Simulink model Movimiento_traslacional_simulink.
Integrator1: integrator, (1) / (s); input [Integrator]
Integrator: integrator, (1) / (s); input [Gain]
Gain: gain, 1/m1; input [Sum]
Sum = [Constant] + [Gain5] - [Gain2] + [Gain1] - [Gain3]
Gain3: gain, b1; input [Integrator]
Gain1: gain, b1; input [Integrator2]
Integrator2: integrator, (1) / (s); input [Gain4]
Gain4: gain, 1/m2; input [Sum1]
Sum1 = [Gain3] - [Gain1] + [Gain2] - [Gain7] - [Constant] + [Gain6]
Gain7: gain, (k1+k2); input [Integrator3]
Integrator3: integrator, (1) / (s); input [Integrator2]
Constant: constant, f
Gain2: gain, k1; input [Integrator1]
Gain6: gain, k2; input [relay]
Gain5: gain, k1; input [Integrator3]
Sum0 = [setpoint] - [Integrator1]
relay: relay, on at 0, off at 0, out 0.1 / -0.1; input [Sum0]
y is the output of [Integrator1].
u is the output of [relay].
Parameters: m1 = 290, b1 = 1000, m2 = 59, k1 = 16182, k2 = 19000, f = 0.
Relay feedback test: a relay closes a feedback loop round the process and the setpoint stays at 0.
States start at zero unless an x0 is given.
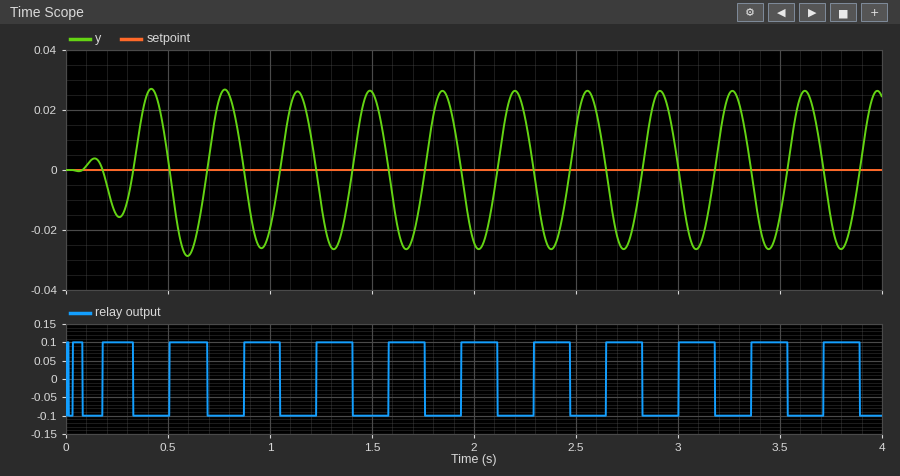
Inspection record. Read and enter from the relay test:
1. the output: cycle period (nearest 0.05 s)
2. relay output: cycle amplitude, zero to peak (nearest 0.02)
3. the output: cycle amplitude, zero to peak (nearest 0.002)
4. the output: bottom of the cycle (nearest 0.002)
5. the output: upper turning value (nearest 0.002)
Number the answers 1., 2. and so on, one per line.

1. 0.35 s
2. 0.10
3. 0.026
4. -0.026
5. 0.026
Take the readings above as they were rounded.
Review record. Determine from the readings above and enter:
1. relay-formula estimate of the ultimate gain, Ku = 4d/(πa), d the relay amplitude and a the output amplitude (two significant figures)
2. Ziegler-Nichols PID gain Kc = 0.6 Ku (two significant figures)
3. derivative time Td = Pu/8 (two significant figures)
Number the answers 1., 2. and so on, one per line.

1. 4.9
2. 2.9
3. 0.044 s
